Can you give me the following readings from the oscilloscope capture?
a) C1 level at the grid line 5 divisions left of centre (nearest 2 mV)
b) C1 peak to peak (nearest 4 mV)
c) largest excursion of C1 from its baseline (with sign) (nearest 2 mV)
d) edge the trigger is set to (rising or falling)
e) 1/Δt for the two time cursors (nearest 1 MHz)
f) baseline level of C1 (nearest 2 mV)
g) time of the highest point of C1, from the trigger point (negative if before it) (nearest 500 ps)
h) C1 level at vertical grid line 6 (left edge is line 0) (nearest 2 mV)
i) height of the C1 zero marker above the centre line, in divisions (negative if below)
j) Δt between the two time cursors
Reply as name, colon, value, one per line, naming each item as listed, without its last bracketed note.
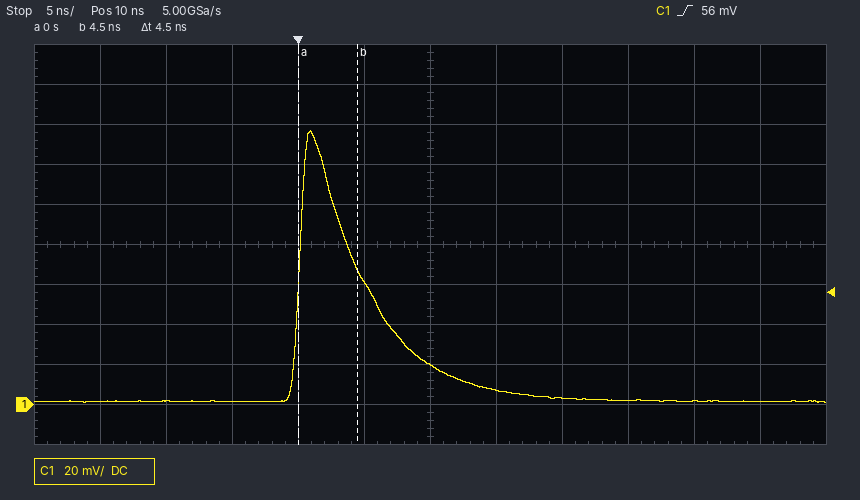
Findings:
C1 level at the grid line 5 divisions left of centre: 2 mV
C1 peak to peak: 136 mV
largest excursion of C1 from its baseline (with sign): +136 mV
edge the trigger is set to: rising
1/Δt for the two time cursors: 222 MHz
baseline level of C1: 2 mV
time of the highest point of C1, from the trigger point (negative if before it): +1.0 ns
C1 level at vertical grid line 6 (left edge is line 0): 20 mV
height of the C1 zero marker above the centre line, in divisions: -4.0 div
Δt between the two time cursors: 4.5 ns
